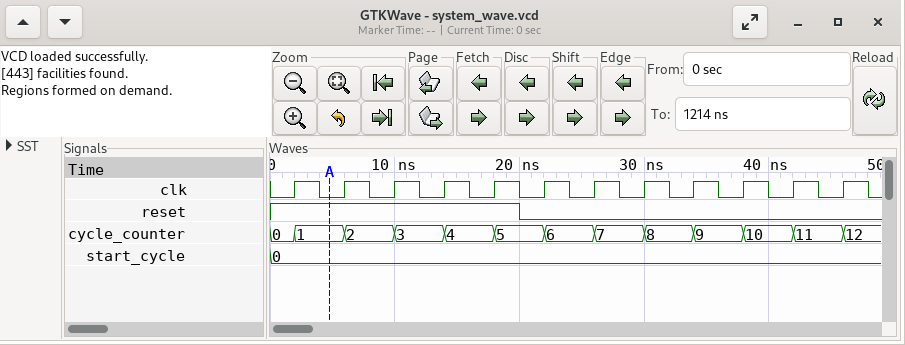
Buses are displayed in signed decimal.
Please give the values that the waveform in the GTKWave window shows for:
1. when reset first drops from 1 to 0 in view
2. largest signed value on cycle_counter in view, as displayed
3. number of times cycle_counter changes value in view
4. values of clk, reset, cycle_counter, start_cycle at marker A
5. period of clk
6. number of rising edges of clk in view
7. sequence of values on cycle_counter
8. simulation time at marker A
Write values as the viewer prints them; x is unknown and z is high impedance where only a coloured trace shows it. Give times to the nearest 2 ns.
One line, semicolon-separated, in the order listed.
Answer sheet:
20 ns; 12; 12; clk=0, reset=1, cycle_counter=1, start_cycle=0; 4 ns; 12; 0, 1, 2, 3, 4, 5, 6, 7, 8, 9, 10, 11, 12; 4 ns
